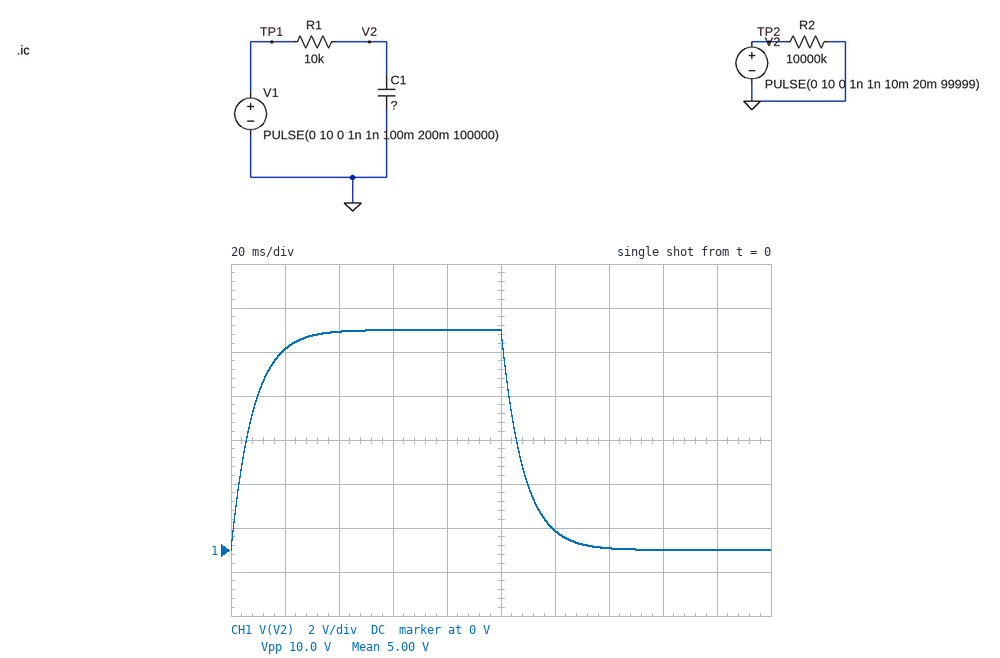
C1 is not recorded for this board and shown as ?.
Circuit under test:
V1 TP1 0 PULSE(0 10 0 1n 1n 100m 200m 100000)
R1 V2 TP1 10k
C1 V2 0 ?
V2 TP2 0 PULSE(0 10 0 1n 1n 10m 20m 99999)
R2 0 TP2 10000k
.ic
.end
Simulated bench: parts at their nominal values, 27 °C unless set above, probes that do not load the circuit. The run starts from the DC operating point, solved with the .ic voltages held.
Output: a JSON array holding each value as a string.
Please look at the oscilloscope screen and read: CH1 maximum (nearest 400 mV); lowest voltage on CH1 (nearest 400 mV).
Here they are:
["10.0 V", "0 V"]
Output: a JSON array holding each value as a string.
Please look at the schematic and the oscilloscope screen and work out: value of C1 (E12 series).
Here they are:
["820 nF"]
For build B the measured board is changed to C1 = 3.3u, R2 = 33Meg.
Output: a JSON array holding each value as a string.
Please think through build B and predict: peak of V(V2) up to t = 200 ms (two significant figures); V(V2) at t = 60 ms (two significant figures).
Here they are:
["9.5 V", "8.4 V"]
